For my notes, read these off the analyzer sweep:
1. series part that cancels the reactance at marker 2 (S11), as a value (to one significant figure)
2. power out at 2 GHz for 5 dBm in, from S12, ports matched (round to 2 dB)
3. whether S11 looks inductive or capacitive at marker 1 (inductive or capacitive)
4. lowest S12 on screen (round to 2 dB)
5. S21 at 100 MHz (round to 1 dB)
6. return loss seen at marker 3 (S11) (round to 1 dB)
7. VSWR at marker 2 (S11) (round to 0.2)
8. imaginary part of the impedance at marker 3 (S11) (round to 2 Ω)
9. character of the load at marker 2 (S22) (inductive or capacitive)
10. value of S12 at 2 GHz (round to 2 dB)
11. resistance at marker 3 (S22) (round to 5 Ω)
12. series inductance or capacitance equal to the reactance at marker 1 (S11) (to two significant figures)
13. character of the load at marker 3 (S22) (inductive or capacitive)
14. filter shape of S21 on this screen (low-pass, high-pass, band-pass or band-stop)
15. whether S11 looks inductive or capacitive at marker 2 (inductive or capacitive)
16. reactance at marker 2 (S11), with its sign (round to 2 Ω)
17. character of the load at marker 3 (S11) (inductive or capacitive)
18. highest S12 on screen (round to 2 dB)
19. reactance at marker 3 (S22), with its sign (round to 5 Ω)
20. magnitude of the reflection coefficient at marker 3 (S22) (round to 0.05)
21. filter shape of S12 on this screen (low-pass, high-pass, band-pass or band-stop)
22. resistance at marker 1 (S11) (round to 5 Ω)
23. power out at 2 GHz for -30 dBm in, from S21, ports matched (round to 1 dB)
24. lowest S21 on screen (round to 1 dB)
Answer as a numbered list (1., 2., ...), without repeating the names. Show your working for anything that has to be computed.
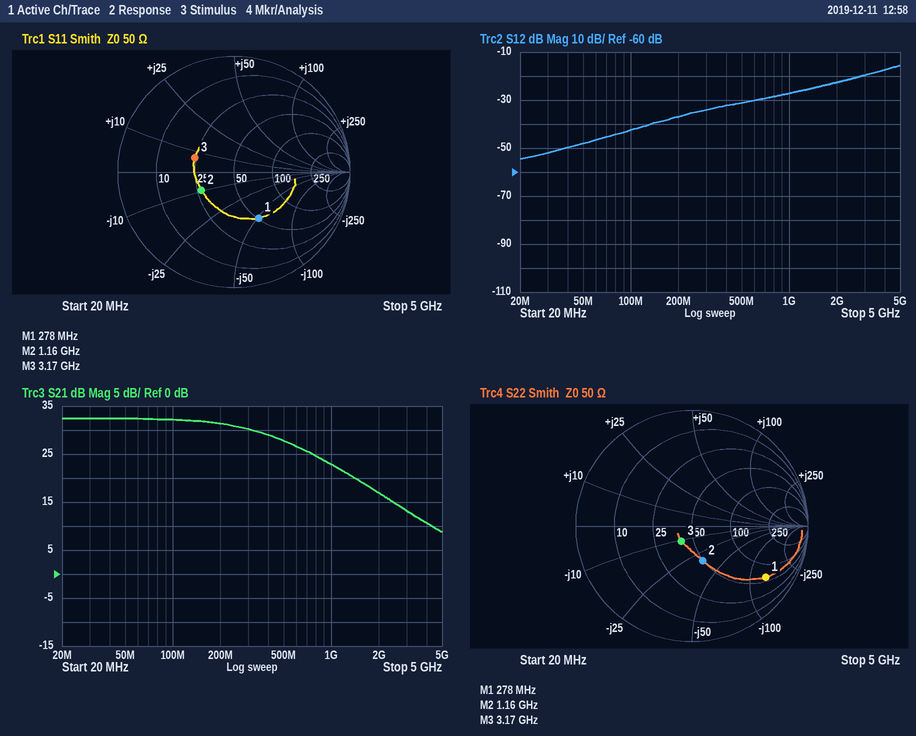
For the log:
1. L = 10 Ω/(2π × 1.16 GHz) ≈ 1 nH
2. 5 dBm + (-22 dB) = -18 dBm
3. capacitive
4. -54 dB
5. 32 dB
6. 9 dB
7. 2.0
8. +6 Ω
9. capacitive
10. -22 dB
11. 40 Ω
12. C = 1/(2π × 278 MHz × 50 Ω) ≈ 11 pF
13. capacitive
14. low-pass
15. capacitive
16. -10 Ω
17. inductive
18. -16 dB
19. -10 Ω
20. 0.15
21. high-pass
22. 50 Ω
23. -30 dBm + (17 dB) = -13 dBm
24. 9 dB
